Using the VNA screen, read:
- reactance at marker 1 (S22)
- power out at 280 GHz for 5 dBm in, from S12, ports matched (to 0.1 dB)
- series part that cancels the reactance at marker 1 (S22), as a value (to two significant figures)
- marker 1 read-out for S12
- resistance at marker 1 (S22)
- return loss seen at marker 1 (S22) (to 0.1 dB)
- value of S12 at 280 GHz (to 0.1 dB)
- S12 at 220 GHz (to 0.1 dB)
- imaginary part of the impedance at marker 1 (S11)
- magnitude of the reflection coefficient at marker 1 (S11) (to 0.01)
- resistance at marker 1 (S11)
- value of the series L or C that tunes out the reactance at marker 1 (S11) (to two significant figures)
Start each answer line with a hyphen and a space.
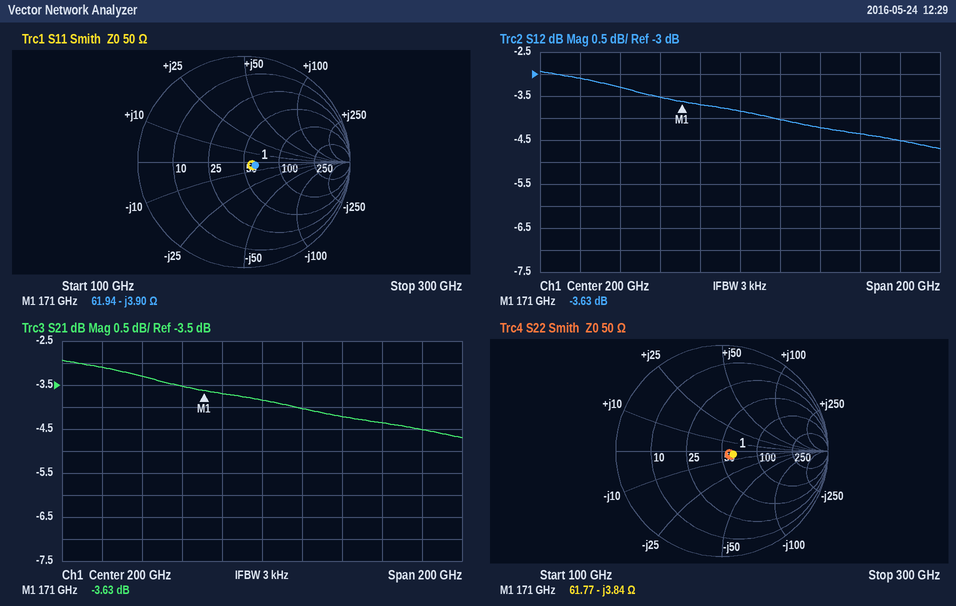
- -3.84 Ω
- 0.5 dBm
- 3.6 pH
- -3.63 dB
- 61.77 Ω
- 19.1 dB
- -4.5 dB
- -4.0 dB
- -3.90 Ω
- 0.11
- 61.94 Ω
- 3.6 pH
